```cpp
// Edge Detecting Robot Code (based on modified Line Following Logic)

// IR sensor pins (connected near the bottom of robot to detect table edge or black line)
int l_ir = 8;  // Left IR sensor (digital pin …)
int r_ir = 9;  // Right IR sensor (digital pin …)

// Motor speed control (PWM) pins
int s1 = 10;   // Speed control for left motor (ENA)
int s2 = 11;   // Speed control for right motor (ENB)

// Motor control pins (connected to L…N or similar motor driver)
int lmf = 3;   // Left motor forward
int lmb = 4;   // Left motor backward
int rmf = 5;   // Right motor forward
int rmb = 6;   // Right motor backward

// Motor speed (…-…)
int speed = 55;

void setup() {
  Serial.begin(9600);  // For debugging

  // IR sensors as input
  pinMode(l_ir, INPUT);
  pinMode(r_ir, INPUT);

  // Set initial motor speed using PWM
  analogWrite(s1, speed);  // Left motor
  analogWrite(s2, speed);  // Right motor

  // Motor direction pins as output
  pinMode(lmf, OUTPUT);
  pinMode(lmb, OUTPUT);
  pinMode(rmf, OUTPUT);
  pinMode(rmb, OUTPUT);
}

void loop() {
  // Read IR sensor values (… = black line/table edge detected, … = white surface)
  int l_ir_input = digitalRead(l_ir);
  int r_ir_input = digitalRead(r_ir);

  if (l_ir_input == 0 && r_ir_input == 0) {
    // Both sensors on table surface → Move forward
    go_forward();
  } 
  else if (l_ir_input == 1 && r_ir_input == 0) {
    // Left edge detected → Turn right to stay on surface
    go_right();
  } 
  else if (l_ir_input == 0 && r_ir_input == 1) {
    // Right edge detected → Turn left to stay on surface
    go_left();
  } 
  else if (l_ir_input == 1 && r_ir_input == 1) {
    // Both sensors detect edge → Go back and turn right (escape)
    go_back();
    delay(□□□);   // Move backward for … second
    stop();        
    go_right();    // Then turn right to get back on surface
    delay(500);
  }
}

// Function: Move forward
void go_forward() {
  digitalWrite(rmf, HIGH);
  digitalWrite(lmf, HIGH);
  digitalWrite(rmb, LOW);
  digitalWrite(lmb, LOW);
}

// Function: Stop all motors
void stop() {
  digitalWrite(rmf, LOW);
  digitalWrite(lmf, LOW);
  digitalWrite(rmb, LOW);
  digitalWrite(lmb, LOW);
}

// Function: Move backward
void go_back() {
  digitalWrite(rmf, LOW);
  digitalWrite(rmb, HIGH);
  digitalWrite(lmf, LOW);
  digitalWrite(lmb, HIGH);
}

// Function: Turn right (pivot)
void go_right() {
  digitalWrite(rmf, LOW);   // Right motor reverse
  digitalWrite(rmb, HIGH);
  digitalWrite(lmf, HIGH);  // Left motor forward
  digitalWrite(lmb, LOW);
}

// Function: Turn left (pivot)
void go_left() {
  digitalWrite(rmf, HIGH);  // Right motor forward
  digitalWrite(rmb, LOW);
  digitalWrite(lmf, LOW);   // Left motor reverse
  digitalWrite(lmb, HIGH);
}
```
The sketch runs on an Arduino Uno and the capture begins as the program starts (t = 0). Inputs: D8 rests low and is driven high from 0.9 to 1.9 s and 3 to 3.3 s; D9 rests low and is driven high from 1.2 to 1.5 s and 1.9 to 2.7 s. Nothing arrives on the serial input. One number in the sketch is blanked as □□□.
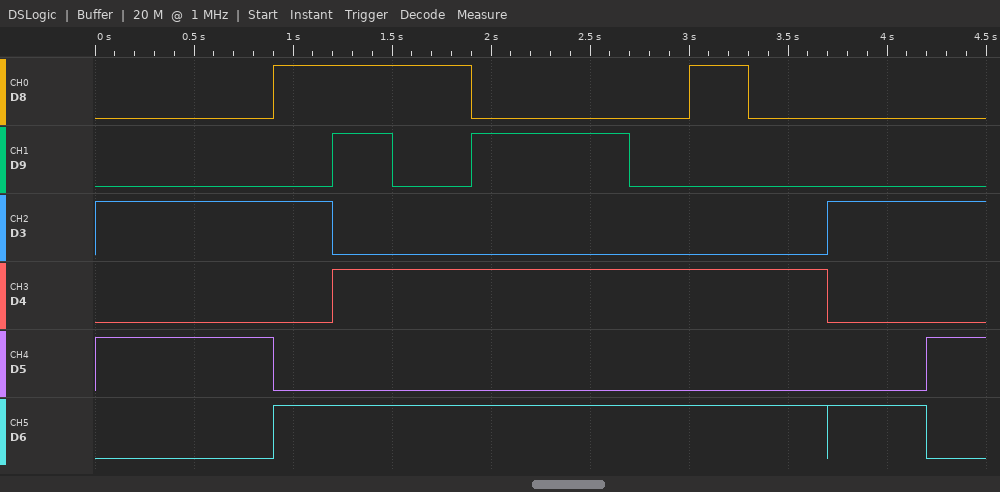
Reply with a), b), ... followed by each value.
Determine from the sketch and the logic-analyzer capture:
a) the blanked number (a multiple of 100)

a) 2500
